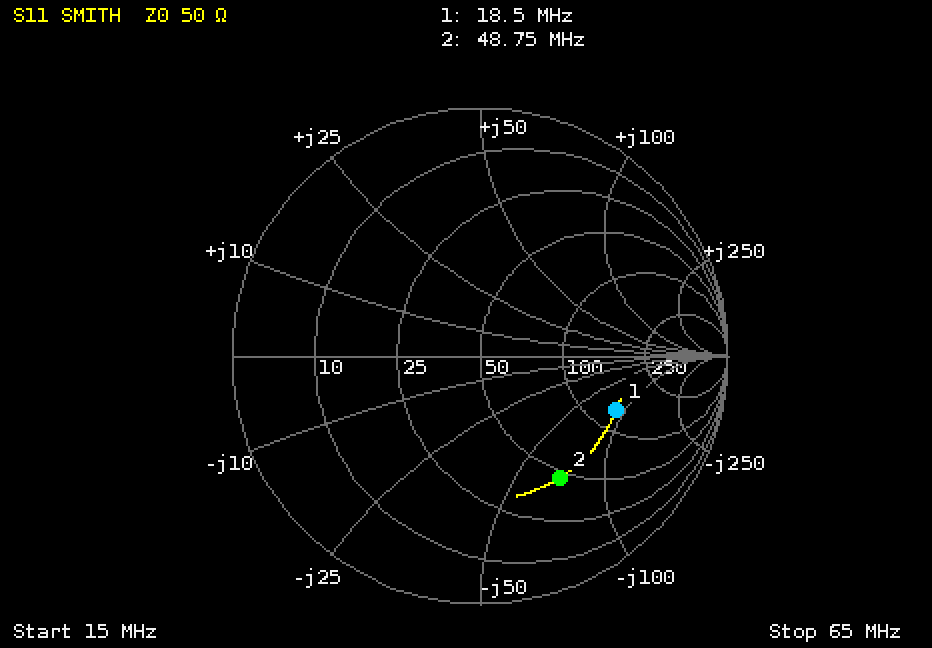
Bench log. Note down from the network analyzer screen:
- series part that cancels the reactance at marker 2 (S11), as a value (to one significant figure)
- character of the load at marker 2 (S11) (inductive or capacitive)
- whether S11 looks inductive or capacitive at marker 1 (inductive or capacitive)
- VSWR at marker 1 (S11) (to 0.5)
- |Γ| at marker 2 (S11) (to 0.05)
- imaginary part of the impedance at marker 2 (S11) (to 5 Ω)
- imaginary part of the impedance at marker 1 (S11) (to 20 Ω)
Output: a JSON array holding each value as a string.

["200 nH", "capacitive", "capacitive", "4.0", "0.60", "-70 Ω", "-80 Ω"]
